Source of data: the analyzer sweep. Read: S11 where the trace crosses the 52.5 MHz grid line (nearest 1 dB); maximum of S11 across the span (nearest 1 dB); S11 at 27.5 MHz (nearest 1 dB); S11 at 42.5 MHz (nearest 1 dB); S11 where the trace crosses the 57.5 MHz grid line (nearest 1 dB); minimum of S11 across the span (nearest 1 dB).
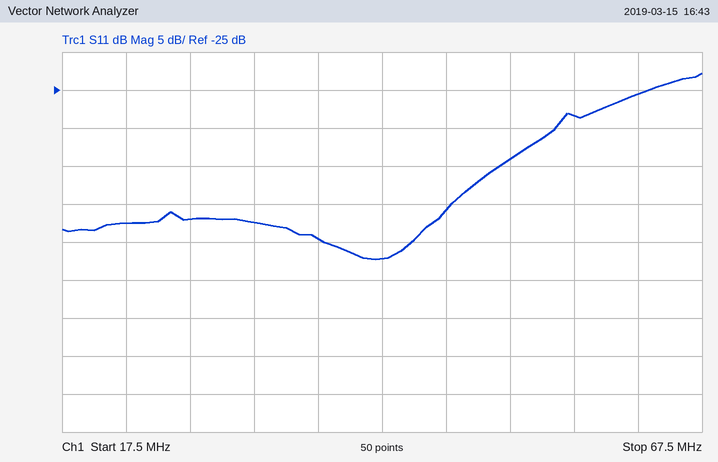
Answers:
-34 dB
-23 dB
-42 dB
-47 dB
-28 dB
-47 dB
